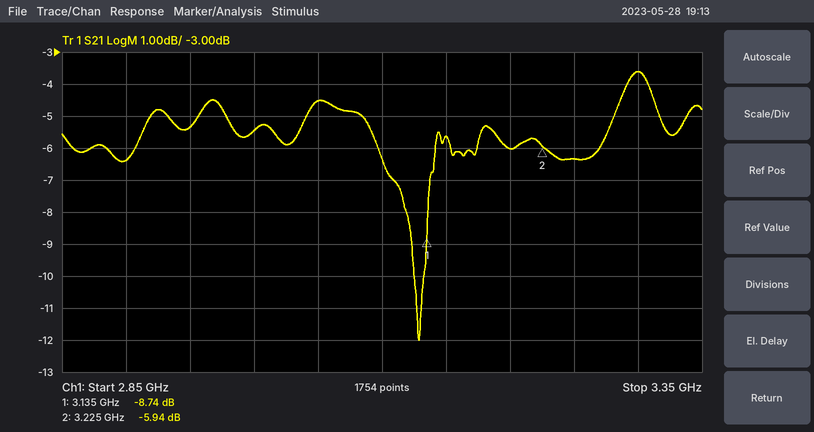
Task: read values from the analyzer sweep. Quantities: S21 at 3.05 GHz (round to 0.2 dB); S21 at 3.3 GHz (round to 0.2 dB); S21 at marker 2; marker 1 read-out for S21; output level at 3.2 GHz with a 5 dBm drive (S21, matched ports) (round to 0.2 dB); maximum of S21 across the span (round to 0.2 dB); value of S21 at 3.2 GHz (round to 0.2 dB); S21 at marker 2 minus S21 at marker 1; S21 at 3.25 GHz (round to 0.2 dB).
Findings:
-4.6 dB
-3.6 dB
-5.94 dB
-8.74 dB
-1.0 dBm
-3.6 dB
-6.0 dB
2.80 dB
-6.4 dB
